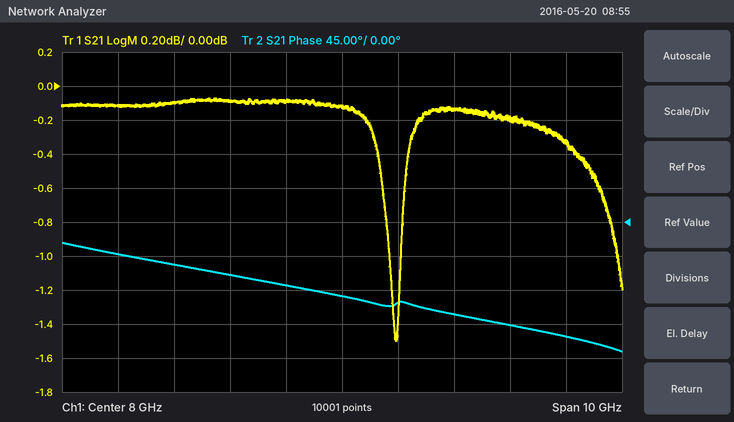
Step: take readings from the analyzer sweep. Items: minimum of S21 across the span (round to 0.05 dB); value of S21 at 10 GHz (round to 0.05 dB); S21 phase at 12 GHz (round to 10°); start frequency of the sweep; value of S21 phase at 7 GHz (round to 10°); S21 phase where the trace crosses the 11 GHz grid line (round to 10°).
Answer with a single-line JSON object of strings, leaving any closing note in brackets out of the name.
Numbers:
{"minimum of S21 across the span": "-1.50 dB", "value of S21 at 10 GHz": "-0.15 dB", "S21 phase at 12 GHz": "-150°", "start frequency of the sweep": "3 GHz", "value of S21 phase at 7 GHz": "-80°", "S21 phase where the trace crosses the 11 GHz grid line": "-140°"}
